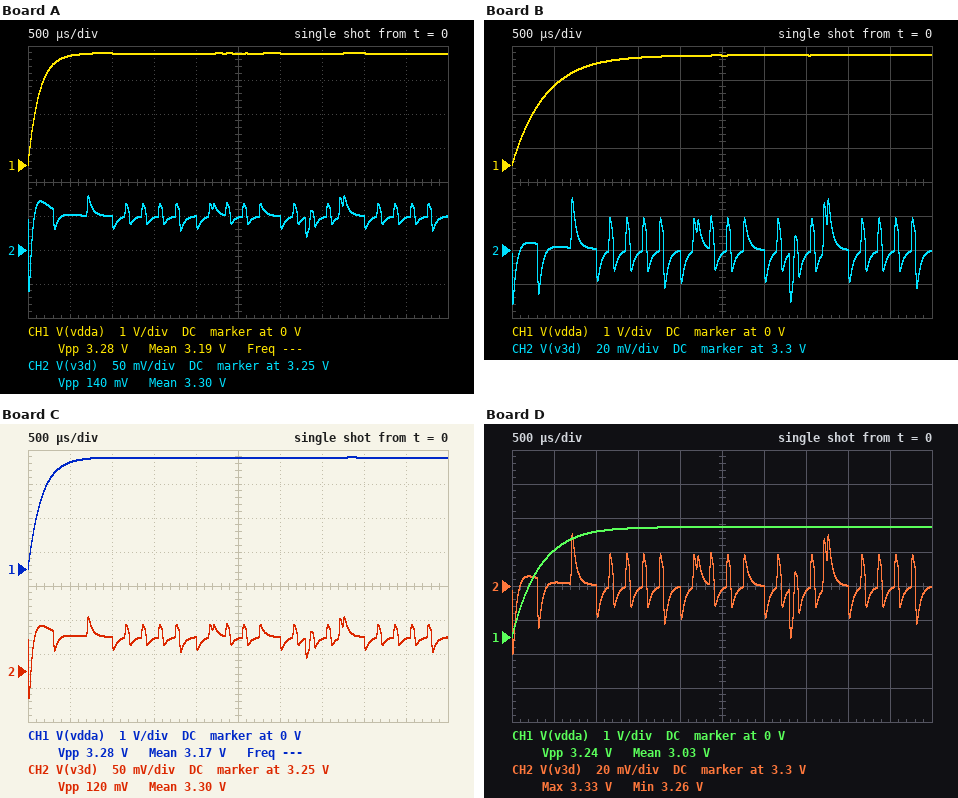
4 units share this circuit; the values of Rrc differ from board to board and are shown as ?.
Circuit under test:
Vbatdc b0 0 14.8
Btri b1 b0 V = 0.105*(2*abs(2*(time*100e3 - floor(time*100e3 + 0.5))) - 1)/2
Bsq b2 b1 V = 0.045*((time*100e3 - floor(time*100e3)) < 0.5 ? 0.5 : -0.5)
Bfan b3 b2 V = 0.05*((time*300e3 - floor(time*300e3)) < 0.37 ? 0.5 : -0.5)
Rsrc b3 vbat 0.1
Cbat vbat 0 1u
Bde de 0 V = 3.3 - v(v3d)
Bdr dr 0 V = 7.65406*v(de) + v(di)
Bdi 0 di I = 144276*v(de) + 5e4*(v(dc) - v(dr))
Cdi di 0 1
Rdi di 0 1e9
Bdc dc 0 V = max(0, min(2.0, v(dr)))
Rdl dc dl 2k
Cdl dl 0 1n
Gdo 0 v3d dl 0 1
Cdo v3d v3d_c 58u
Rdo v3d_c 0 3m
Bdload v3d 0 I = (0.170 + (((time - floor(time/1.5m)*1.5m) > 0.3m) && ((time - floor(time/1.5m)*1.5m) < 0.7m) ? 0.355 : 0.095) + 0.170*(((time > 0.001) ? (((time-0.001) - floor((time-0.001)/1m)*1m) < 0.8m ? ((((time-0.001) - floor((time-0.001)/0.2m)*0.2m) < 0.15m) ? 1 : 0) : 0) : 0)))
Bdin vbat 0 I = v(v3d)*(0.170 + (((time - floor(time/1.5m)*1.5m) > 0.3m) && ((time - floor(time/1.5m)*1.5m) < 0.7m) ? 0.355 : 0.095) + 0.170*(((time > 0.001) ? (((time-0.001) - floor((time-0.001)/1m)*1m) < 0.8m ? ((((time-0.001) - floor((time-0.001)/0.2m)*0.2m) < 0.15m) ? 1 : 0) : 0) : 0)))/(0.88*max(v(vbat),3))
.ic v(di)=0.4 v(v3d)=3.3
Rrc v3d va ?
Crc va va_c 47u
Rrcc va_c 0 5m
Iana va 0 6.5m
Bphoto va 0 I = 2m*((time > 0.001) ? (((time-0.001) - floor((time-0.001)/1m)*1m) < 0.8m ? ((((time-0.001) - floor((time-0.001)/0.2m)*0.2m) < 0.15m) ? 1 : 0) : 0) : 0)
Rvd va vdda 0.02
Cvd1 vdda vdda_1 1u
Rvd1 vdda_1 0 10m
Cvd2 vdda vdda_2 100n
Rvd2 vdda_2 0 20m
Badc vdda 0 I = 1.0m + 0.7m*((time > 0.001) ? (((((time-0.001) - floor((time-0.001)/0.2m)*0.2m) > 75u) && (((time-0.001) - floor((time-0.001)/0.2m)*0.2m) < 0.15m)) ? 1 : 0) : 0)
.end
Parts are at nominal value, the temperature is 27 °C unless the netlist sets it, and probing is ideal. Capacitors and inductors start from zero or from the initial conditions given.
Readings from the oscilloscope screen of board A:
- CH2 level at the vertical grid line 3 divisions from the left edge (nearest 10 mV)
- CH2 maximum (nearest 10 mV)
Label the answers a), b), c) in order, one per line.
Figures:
a) 3.30 V
b) 3.33 V
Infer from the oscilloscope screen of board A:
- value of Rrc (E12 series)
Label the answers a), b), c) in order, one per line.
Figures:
a) 2.7 Ω
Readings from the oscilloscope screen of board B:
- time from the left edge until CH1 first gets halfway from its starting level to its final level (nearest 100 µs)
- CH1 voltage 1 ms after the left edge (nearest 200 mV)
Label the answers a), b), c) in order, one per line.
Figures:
a) 300 µs
b) 3.0 V
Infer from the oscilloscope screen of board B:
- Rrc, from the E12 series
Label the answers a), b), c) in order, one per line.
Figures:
a) 8.2 Ω
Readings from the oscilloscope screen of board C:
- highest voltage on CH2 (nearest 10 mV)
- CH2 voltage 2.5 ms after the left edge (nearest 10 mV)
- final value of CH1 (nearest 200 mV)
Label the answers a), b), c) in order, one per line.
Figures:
a) 3.33 V
b) 3.30 V
c) 3.2 V
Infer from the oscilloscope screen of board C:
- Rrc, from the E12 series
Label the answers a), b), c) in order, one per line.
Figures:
a) 3.3 Ω
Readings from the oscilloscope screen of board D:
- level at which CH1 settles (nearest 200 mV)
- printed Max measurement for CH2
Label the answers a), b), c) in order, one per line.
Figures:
a) 3.2 V
b) 3.33 V
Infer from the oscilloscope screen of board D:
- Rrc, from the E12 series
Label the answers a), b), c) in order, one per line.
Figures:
a) 6.8 Ω
